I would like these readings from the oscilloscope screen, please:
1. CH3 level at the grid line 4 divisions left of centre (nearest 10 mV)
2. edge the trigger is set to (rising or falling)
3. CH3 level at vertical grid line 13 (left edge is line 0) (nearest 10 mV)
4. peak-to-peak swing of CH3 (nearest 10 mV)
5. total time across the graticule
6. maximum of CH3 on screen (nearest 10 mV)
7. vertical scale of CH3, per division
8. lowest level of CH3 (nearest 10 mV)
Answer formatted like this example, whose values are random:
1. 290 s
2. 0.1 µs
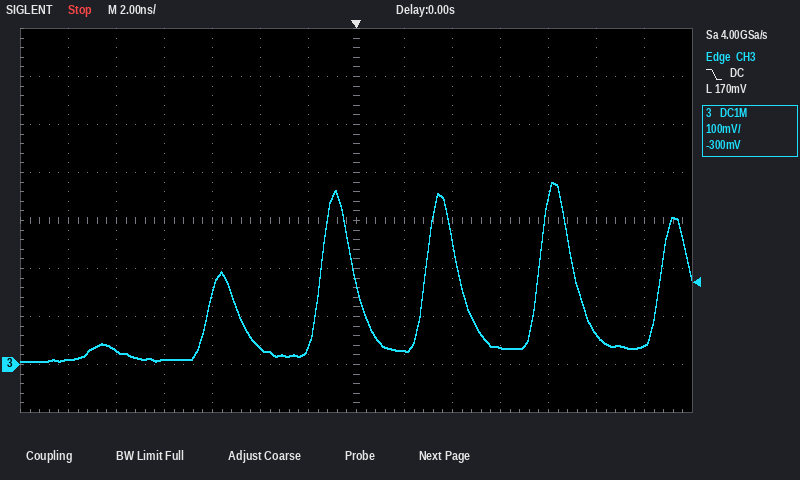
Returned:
1. 10 mV
2. falling
3. 40 mV
4. 370 mV
5. 28 ns
6. 380 mV
7. 100 mV
8. 10 mV
